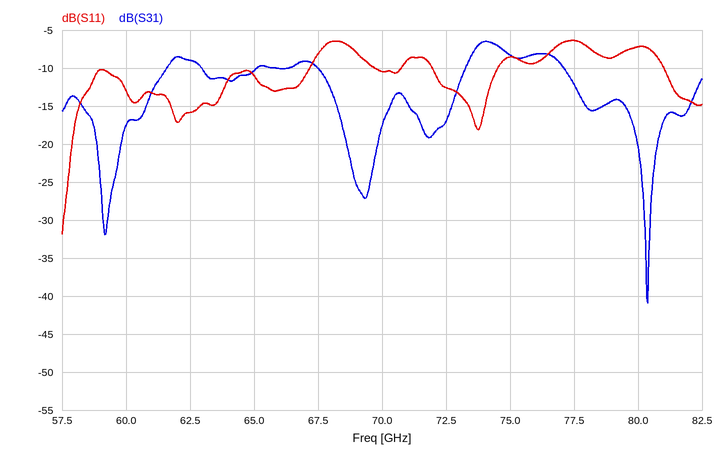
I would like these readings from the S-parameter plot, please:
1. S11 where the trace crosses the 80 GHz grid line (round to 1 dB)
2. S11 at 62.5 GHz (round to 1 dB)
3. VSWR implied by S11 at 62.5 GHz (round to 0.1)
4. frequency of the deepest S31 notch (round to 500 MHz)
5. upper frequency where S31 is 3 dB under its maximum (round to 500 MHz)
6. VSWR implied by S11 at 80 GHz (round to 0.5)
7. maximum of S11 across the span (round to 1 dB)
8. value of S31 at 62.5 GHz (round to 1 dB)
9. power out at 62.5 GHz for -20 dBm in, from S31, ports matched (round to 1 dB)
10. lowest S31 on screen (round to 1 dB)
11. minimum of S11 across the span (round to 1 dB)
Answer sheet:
-7 dB
-16 dB
1.4
80.5 GHz
77.0 GHz
2.5
-6 dB
-9 dB
-29 dBm
-41 dB
-32 dB
